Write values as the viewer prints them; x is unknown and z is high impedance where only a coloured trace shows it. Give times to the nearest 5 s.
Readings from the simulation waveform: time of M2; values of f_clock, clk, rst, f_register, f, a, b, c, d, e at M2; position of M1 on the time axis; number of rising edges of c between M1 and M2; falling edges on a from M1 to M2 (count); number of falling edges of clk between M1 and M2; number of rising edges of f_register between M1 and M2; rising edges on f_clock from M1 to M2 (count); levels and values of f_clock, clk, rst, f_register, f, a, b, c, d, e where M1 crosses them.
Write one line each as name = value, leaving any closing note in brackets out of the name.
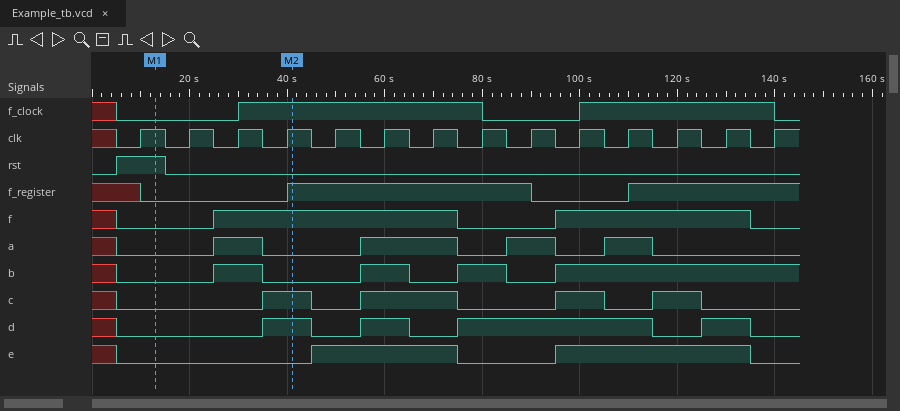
time of M2 = 40 s
values of f_clock, clk, rst, f_register, f, a, b, c, d, e at M2 = f_clock=1, clk=1, rst=0, f_register=1, f=1, a=0, b=0, c=1, d=1, e=0
position of M1 on the time axis = 15 s
number of rising edges of c between M1 and M2 = 1
falling edges on a from M1 to M2 = 1
number of falling edges of clk between M1 and M2 = 3
number of rising edges of f_register between M1 and M2 = 1
rising edges on f_clock from M1 to M2 = 1
levels and values of f_clock, clk, rst, f_register, f, a, b, c, d, e where M1 crosses them = f_clock=0, clk=1, rst=1, f_register=0, f=0, a=0, b=0, c=0, d=0, e=0
